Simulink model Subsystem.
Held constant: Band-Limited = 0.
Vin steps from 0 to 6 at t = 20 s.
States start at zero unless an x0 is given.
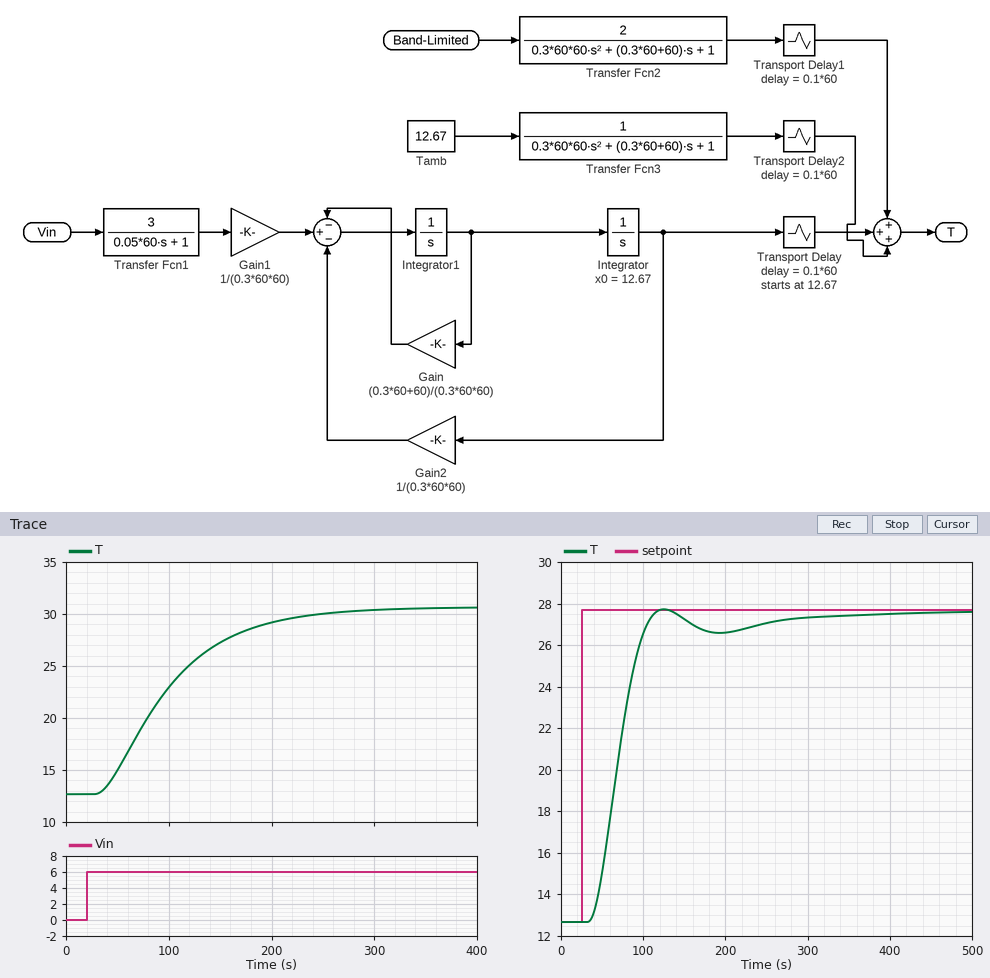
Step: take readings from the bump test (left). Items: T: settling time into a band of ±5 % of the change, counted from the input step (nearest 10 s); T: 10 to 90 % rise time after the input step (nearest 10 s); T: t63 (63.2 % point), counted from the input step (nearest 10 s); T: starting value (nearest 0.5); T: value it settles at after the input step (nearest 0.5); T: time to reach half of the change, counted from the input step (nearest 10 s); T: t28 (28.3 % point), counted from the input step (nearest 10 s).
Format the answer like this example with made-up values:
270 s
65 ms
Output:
210 s
140 s
90 s
12.5
30.5
70 s
50 s
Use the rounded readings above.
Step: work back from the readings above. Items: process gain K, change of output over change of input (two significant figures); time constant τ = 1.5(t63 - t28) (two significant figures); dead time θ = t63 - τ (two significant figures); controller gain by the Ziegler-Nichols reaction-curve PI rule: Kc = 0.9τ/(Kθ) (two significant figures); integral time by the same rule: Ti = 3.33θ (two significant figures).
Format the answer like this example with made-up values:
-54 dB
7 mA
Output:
3.0
60 s
30 s
0.60
100 s
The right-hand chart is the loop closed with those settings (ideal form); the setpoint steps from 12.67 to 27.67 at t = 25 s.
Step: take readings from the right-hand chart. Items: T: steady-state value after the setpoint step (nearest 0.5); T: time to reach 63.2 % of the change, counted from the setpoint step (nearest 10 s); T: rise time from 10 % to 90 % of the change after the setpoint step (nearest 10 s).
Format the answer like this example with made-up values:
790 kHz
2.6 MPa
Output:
27.5
50 s
50 s
